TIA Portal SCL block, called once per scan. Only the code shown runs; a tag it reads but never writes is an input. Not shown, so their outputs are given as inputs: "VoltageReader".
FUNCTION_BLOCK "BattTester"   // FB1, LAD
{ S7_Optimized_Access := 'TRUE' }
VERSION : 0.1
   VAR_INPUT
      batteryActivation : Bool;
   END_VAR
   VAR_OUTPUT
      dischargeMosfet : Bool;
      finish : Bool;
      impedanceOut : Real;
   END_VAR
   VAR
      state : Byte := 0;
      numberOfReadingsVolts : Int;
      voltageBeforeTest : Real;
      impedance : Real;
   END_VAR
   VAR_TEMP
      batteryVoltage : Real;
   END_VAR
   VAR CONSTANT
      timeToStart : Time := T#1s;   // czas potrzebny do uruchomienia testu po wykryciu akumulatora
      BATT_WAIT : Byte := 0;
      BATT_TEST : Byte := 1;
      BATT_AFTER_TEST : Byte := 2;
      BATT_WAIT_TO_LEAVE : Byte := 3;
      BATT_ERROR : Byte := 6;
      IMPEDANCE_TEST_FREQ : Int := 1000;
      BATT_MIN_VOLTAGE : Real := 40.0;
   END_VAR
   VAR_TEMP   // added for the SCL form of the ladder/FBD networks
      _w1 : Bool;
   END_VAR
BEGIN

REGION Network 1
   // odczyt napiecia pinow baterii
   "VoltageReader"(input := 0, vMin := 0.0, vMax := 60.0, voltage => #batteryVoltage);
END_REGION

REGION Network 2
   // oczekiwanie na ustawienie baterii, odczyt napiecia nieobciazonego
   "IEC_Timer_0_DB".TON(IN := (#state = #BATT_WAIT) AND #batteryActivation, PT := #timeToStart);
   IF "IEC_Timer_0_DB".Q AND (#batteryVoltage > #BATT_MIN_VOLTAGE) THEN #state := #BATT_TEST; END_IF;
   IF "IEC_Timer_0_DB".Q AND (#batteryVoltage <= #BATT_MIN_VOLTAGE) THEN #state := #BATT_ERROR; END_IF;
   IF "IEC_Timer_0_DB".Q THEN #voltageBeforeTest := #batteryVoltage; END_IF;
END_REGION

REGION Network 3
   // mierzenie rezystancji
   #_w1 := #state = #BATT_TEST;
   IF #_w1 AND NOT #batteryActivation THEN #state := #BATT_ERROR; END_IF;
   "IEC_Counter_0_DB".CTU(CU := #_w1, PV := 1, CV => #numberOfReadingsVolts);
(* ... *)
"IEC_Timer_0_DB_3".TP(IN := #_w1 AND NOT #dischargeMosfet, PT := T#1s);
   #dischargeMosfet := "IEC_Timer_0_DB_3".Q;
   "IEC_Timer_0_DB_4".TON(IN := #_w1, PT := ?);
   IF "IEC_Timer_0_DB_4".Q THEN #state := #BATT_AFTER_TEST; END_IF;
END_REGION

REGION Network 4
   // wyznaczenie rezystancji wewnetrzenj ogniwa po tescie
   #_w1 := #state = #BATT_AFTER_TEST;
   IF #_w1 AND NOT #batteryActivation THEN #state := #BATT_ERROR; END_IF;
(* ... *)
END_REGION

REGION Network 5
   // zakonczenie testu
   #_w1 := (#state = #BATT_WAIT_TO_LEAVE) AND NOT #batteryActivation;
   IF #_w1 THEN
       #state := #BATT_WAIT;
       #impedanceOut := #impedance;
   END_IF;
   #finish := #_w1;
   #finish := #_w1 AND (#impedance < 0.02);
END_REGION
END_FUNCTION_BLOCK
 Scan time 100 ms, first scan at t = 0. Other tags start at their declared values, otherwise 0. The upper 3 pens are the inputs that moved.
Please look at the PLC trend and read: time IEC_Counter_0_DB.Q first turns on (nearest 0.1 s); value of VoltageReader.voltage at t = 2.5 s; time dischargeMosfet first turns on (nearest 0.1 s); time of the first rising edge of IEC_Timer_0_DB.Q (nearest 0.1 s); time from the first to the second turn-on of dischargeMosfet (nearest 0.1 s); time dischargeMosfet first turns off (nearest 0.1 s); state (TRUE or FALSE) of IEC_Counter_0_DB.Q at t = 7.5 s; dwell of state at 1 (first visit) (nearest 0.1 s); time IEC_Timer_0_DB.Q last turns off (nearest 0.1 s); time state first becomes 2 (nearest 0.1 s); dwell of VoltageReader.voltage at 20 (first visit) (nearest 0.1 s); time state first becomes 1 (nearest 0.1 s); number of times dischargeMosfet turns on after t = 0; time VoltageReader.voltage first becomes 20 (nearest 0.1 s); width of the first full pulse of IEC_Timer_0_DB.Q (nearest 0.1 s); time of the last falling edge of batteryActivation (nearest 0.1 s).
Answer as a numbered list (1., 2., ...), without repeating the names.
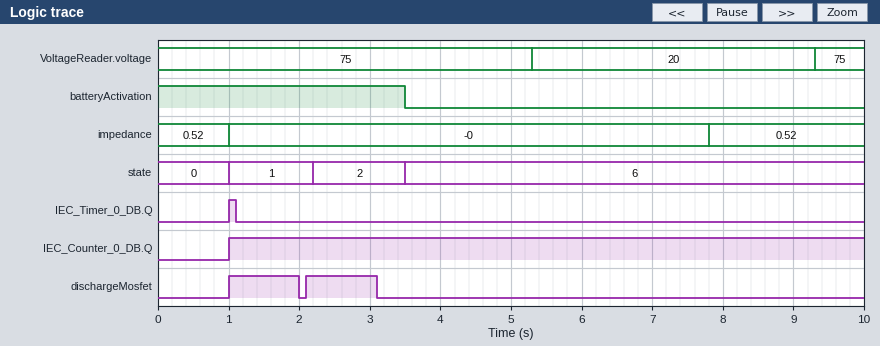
1. 1.0 s
2. 75
3. 1.0 s
4. 1.0 s
5. 1.1 s
6. 2.0 s
7. TRUE
8. 1.2 s
9. 1.1 s
10. 2.2 s
11. 4.0 s
12. 1.0 s
13. 2
14. 5.3 s
15. 0.1 s
16. 3.5 s
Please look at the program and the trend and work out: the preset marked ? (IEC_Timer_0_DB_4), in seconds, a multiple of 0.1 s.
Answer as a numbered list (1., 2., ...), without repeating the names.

1. 1.2 s
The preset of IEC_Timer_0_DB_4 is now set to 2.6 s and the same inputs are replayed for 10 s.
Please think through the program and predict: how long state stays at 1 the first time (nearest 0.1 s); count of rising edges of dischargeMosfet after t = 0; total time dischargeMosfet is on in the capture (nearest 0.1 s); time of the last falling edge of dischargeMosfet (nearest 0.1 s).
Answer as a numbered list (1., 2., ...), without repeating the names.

1. 2.5 s
2. 3
3. 3.0 s
4. 4.2 s
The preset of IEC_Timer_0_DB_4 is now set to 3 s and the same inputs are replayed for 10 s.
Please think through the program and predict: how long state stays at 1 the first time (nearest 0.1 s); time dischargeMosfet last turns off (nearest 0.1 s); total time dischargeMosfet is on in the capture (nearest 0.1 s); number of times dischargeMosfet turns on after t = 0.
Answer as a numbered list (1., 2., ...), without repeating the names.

1. 2.5 s
2. 4.2 s
3. 3.0 s
4. 3
